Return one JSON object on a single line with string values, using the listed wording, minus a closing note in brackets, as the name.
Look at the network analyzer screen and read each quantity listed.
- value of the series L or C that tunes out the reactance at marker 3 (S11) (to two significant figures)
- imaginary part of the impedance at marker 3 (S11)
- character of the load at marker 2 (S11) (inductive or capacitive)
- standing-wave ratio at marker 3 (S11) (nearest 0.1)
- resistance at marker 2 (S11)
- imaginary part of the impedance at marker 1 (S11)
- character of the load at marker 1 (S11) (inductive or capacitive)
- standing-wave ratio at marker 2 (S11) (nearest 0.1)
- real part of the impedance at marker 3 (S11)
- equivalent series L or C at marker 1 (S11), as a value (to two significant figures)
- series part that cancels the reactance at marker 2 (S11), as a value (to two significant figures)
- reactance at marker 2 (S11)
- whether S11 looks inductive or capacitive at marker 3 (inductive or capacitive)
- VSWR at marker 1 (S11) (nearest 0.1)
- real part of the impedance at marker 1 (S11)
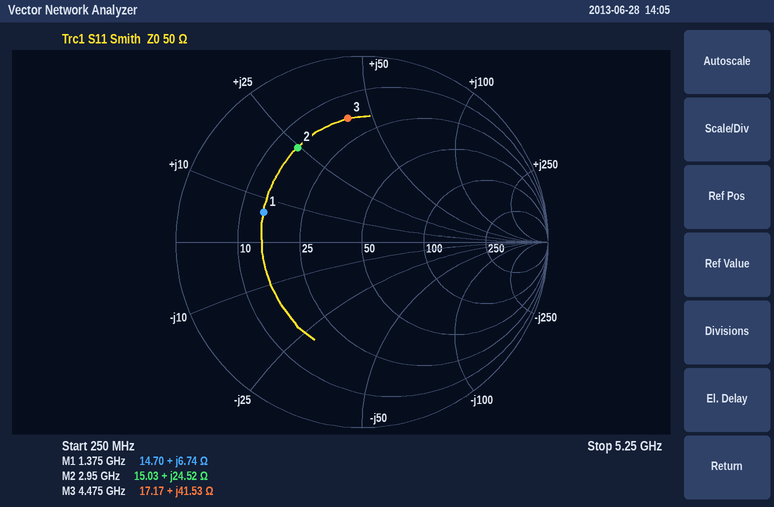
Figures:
{"value of the series L or C that tunes out the reactance at marker 3 (S11)": "860 fF", "imaginary part of the impedance at marker 3": "+41.53 Ω", "character of the load at marker 2 (S11)": "inductive", "standing-wave ratio at marker 3 (S11)": "5.1", "resistance at marker 2": "15.03 Ω", "imaginary part of the impedance at marker 1": "+6.74 Ω", "character of the load at marker 1 (S11)": "inductive", "standing-wave ratio at marker 2 (S11)": "4.2", "real part of the impedance at marker 3": "17.17 Ω", "equivalent series L or C at marker 1 (S11), as a value": "780 pH", "series part that cancels the reactance at marker 2 (S11), as a value": "2.2 pF", "reactance at marker 2": "+24.52 Ω", "whether S11 looks inductive or capacitive at marker 3": "inductive", "VSWR at marker 1 (S11)": "3.5", "real part of the impedance at marker 1": "14.70 Ω"}
